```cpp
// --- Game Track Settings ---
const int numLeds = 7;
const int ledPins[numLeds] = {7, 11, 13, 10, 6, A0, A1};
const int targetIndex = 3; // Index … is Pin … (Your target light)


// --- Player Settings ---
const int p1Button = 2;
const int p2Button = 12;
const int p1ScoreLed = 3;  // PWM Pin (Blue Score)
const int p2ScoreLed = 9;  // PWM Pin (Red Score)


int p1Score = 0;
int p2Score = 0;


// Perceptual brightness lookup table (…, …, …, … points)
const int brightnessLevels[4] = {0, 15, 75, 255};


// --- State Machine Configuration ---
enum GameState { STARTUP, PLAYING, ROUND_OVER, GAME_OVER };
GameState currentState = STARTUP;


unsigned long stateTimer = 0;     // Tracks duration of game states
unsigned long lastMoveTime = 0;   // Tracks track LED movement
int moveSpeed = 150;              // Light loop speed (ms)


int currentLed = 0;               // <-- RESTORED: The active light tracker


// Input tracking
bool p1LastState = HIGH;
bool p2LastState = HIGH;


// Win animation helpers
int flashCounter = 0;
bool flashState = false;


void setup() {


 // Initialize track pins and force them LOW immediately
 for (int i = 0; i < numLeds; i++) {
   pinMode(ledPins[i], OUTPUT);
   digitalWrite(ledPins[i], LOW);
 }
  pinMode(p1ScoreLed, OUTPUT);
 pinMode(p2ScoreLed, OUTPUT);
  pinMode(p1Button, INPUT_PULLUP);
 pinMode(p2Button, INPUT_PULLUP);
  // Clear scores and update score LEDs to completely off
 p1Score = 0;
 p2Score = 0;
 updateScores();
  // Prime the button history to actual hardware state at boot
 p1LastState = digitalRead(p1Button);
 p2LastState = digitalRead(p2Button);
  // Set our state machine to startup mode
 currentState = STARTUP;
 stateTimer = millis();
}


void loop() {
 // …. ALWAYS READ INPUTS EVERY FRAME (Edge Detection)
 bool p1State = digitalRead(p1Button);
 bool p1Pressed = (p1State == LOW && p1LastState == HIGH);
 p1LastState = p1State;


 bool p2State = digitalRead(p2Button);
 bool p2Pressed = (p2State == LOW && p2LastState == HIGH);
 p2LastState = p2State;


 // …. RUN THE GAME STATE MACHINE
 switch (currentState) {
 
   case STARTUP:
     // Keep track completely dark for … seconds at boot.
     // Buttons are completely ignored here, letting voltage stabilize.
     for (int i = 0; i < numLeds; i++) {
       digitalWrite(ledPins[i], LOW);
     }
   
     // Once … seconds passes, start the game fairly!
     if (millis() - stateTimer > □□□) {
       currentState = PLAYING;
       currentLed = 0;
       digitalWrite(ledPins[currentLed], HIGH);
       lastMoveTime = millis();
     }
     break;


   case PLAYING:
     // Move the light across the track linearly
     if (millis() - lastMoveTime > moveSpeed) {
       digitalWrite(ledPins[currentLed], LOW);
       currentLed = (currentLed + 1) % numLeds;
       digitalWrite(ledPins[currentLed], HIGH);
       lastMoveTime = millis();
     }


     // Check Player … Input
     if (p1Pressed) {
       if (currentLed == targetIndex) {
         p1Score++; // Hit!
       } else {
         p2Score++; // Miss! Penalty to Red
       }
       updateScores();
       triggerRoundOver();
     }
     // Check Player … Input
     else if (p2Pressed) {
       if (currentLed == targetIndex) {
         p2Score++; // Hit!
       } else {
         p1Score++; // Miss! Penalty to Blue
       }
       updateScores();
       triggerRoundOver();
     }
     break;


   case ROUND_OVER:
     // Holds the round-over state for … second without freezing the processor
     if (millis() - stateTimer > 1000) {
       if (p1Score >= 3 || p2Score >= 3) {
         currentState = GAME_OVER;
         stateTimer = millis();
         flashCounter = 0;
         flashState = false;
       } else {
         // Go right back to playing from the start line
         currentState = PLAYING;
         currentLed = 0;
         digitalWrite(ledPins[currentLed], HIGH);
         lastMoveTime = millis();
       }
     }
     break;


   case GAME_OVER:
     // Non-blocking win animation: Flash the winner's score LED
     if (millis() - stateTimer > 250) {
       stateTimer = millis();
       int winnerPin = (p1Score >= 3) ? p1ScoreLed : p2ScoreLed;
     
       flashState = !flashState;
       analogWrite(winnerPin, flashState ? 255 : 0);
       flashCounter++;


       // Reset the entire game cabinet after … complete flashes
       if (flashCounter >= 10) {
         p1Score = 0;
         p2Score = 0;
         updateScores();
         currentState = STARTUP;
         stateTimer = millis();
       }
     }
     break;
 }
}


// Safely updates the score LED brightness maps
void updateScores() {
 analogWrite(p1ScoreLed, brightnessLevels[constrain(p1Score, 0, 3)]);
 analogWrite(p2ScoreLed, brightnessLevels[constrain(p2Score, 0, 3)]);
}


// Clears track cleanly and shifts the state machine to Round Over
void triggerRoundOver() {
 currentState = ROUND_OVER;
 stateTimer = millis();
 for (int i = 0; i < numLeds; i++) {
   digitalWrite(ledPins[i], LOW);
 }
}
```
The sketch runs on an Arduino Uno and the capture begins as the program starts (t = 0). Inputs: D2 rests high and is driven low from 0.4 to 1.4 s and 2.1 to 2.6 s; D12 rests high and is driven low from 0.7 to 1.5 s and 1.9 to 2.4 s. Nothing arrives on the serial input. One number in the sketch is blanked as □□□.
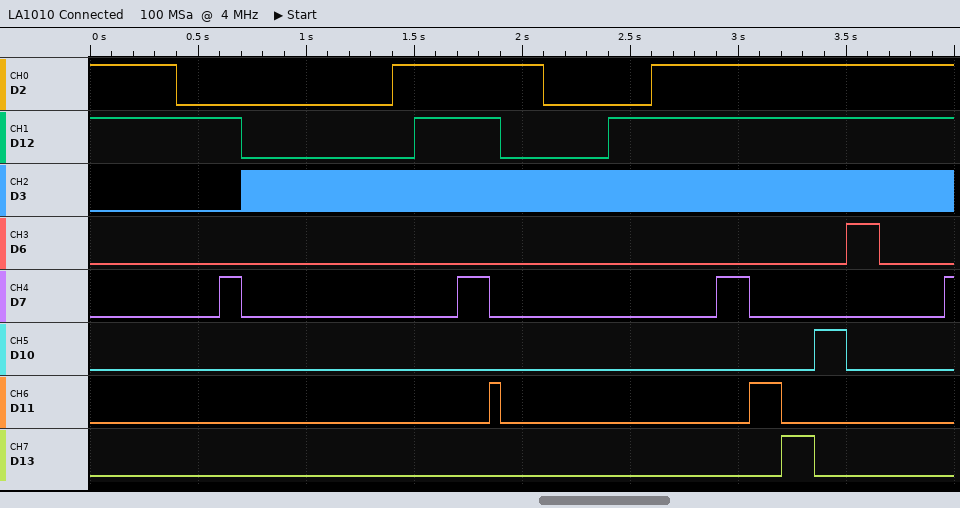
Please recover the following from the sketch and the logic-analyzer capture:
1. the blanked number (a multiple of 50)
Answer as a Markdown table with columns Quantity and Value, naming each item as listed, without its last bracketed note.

| Quantity | Value |
|---|---|
| the blanked number | 600 |
